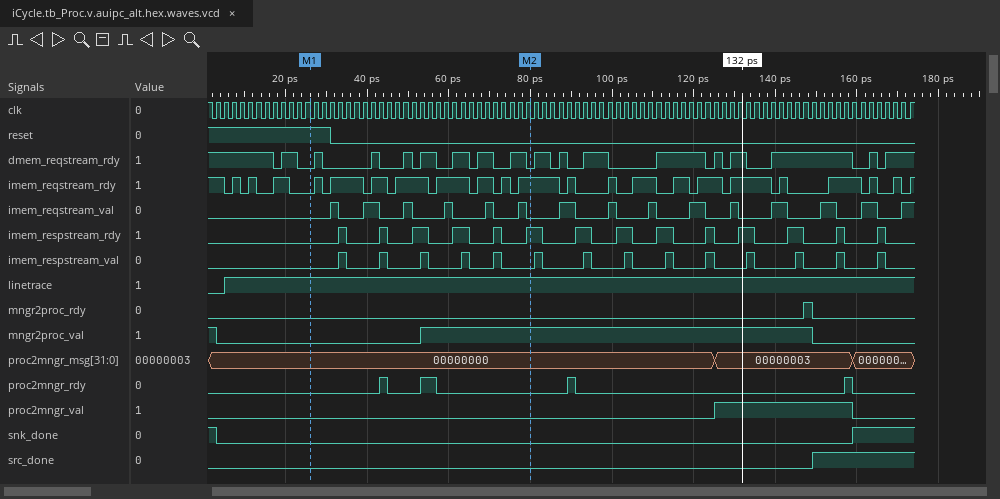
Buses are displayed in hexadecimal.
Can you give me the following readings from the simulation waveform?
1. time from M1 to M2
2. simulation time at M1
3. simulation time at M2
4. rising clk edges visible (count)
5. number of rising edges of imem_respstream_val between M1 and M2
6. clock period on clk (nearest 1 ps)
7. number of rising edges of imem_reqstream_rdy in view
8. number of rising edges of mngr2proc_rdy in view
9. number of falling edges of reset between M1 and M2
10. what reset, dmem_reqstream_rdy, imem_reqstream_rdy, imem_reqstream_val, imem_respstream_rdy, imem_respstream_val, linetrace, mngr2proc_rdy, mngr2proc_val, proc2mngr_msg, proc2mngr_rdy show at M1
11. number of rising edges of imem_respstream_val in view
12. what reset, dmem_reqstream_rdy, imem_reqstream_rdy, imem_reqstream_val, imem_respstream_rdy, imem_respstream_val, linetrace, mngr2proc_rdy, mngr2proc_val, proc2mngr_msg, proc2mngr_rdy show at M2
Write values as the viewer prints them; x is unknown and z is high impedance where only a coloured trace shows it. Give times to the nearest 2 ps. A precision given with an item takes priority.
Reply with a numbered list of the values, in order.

1. 54 ps
2. 26 ps
3. 80 ps
4. 86
5. 5
6. 2 ps
7. 22
8. 1
9. 1
10. reset=1, dmem_reqstream_rdy=0, imem_reqstream_rdy=0, imem_reqstream_val=0, imem_respstream_rdy=0, imem_respstream_val=0, linetrace=1, mngr2proc_rdy=0, mngr2proc_val=0, proc2mngr_msg=00000000, proc2mngr_rdy=0
11. 14
12. reset=0, dmem_reqstream_rdy=0, imem_reqstream_rdy=1, imem_reqstream_val=0, imem_respstream_rdy=1, imem_respstream_val=0, linetrace=1, mngr2proc_rdy=0, mngr2proc_val=1, proc2mngr_msg=00000000, proc2mngr_rdy=0
